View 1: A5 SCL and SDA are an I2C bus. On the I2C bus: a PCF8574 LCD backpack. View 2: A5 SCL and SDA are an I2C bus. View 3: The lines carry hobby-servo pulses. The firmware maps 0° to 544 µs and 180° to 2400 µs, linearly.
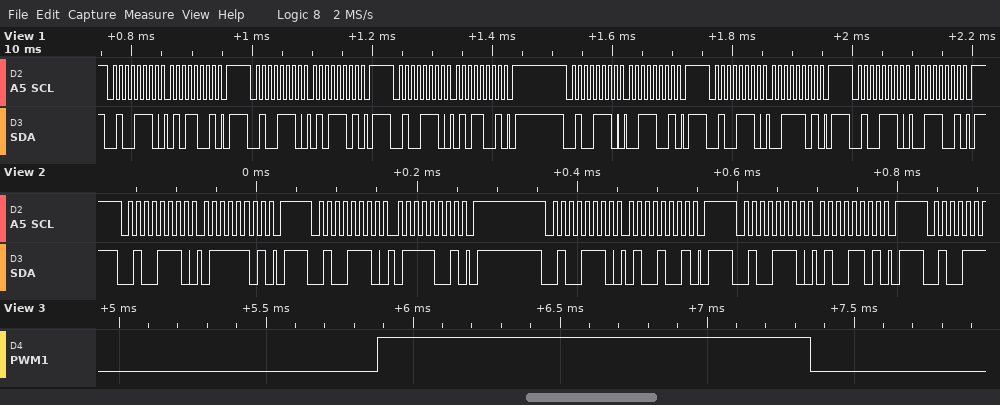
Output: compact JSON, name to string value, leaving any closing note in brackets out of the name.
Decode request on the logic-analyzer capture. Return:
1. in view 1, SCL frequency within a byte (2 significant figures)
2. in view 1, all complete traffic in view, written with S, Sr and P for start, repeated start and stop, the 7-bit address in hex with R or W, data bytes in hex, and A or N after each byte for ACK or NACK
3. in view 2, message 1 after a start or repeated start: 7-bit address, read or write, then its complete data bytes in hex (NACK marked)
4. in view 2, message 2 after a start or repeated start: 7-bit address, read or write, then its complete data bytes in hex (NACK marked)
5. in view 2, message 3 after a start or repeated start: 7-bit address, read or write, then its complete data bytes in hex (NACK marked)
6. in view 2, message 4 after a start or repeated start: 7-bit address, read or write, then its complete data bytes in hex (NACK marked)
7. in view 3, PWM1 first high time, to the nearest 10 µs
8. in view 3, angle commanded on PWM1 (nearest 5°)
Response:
{"in view 1, SCL frequency within a byte": "100 kHz", "in view 1, all complete traffic in view, written with S, Sr and P for start, repeated start and stop, the 7-bit address in hex with R or W, data bytes in hex, and A or N after each byte for ACK or NACK": "S 27W A 59 A P S 27W A 5D A P S 27W A 59 A P S 27W A 39 A P S 27W A 3D A P S 27W A 39 A P", "in view 2, message 1 after a start or repeated start: 7-bit address, read or write, then its complete data bytes in hex": "0x27 write: 7D", "in view 2, message 2 after a start or repeated start: 7-bit address, read or write, then its complete data bytes in hex": "0x27 write: 79", "in view 2, message 3 after a start or repeated start: 7-bit address, read or write, then its complete data bytes in hex": "0x27 write: 49", "in view 2, message 4 after a start or repeated start: 7-bit address, read or write, then its complete data bytes in hex": "0x27 write: 4D", "in view 3, PWM1 first high time, to the nearest 10 µs": "1470 µs", "in view 3, angle commanded on PWM1": "90°"}
